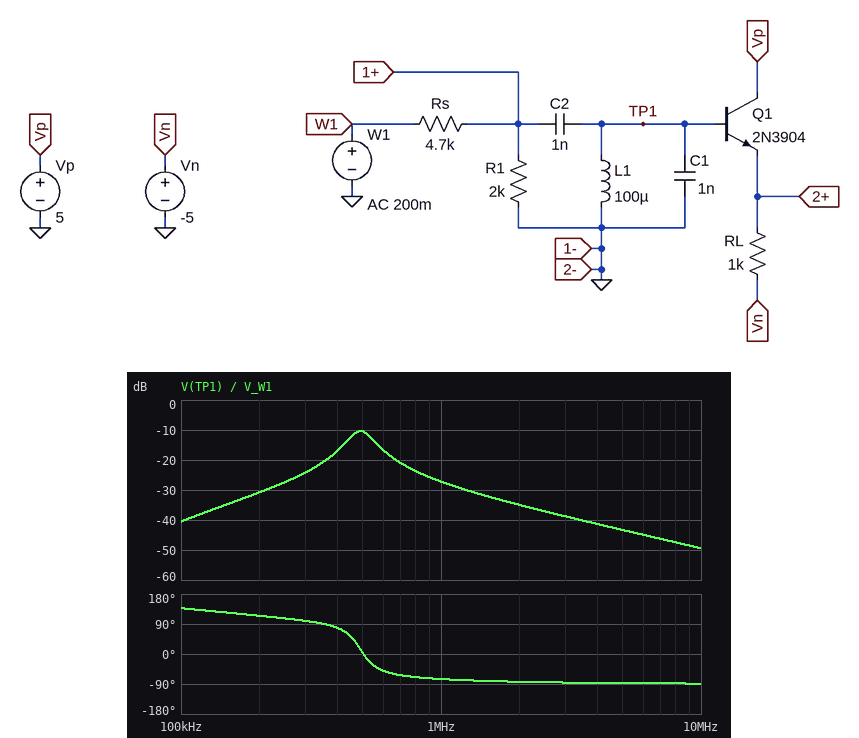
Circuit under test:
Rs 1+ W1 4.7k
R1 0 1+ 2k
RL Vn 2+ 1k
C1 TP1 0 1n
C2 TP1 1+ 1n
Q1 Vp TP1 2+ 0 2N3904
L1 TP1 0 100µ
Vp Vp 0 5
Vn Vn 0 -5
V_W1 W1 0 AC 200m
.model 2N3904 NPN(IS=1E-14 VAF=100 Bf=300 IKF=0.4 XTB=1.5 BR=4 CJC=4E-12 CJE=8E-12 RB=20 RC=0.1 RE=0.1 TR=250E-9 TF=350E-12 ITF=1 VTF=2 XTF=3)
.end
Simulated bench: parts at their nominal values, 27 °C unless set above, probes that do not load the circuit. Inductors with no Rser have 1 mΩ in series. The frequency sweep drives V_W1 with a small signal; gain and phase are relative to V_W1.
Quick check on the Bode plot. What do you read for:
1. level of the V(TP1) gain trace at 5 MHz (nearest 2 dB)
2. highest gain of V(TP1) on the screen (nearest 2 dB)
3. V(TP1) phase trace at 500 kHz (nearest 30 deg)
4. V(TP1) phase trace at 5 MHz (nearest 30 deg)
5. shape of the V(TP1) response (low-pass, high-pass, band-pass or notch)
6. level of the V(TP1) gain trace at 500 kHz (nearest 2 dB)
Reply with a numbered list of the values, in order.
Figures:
1. -44 dB
2. -10 dB
3. 0 deg
4. -90 deg
5. band-pass
6. -10 dB
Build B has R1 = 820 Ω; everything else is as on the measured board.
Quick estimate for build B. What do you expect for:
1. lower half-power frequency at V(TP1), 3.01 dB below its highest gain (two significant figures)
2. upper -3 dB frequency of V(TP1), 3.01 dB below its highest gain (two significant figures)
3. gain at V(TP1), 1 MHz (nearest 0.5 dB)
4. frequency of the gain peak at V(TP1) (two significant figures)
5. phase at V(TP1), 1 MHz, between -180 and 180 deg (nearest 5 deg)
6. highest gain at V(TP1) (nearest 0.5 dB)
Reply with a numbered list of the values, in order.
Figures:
1. 380 kHz
2. 560 kHz
3. -28.0 dB
4. 460 kHz
5. -60 deg
6. -15.5 dB
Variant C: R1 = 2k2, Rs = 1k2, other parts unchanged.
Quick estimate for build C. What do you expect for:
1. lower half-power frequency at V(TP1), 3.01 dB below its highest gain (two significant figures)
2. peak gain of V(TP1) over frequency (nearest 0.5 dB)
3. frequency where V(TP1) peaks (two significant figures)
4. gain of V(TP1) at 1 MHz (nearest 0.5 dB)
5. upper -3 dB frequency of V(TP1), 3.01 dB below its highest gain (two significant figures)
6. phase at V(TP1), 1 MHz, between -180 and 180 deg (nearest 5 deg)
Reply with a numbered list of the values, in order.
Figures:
1. 390 kHz
2. -3.0 dB
3. 460 kHz
4. -16.0 dB
5. 560 kHz
6. -65 deg
